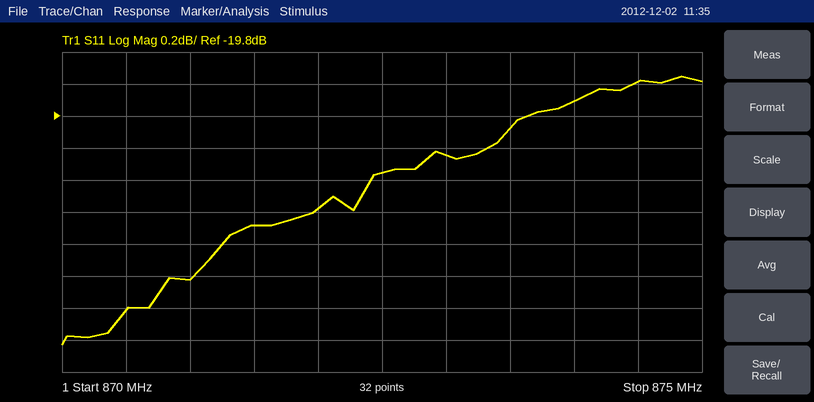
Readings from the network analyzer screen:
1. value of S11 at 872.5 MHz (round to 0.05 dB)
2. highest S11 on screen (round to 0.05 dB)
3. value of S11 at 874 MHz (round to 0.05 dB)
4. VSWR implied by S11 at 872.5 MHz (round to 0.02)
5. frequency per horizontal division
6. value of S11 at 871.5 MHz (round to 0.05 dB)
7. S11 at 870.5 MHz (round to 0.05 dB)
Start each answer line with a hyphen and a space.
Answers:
- -20.15 dB
- -19.55 dB
- -19.70 dB
- 1.22
- 500 kHz
- -20.50 dB
- -21.00 dB
